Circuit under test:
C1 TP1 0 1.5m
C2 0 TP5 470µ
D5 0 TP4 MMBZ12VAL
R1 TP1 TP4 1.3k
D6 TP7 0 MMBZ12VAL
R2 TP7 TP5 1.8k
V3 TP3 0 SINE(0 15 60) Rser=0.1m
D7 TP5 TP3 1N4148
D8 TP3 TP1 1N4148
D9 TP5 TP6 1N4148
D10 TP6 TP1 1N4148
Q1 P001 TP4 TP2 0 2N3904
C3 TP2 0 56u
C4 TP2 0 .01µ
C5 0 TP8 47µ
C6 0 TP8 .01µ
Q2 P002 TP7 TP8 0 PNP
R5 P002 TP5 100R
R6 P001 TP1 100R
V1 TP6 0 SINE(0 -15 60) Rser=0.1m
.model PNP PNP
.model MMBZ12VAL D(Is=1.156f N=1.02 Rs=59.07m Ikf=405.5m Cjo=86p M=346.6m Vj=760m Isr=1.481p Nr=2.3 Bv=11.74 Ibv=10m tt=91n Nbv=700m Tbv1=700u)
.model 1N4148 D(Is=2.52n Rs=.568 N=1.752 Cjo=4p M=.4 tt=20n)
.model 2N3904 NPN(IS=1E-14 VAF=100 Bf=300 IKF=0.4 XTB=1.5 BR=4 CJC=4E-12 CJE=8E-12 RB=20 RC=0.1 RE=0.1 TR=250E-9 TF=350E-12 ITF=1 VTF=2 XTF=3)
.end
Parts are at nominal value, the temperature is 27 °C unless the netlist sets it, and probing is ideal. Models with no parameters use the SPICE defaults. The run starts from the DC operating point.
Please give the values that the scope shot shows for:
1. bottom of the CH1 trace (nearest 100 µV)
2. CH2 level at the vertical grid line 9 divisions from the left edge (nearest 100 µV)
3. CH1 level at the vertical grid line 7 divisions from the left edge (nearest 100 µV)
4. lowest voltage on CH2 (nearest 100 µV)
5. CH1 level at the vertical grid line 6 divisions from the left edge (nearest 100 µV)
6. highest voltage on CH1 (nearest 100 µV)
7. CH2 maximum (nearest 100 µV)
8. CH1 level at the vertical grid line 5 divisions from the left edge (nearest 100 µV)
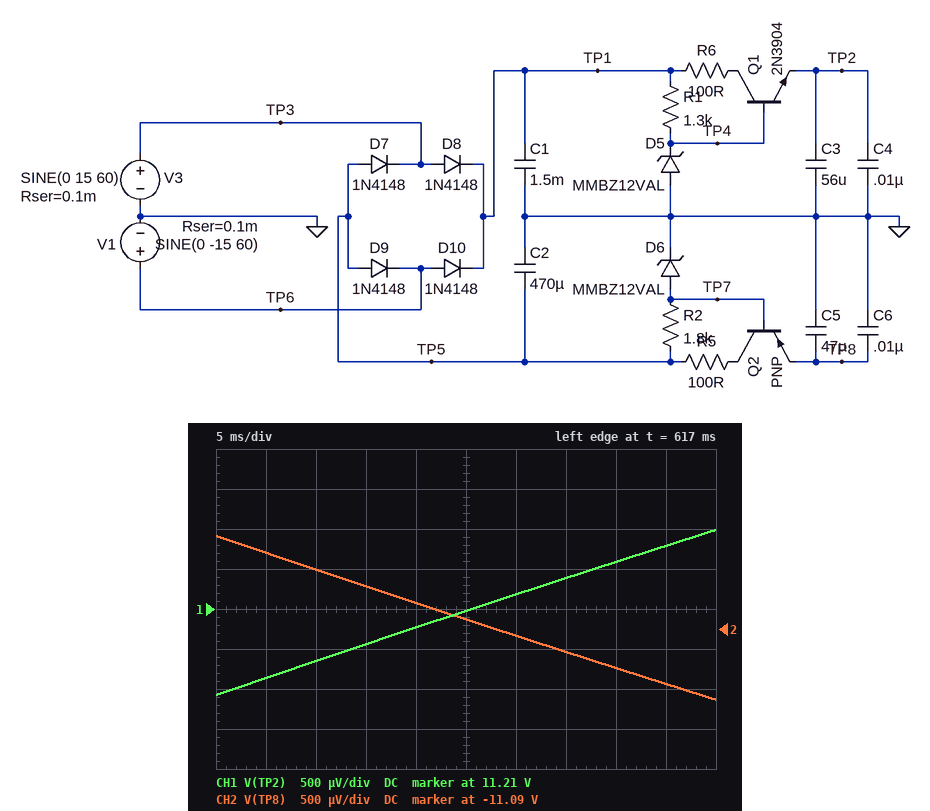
11.2119 V
-11.0932 V
11.2134 V
-11.0934 V
11.2132 V
11.2140 V
-11.0913 V
11.2130 V
